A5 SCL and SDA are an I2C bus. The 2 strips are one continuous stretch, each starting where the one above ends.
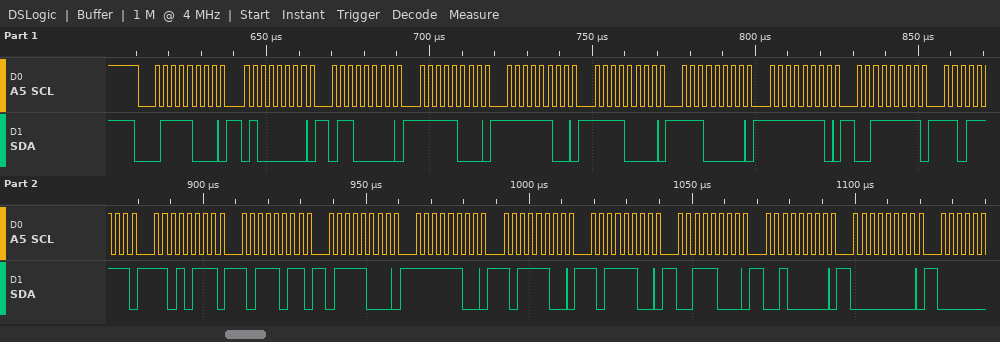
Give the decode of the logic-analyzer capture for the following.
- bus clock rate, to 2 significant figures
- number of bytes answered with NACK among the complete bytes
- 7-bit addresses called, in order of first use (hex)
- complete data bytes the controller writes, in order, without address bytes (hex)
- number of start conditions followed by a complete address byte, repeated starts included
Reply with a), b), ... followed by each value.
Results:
a) 400 kHz
b) 0
c) 0x3C
d) 40 60 F8 FC F0 E0 FE 3F DF D7 BB 78 FC BC BC 38 20 00
e) 1
